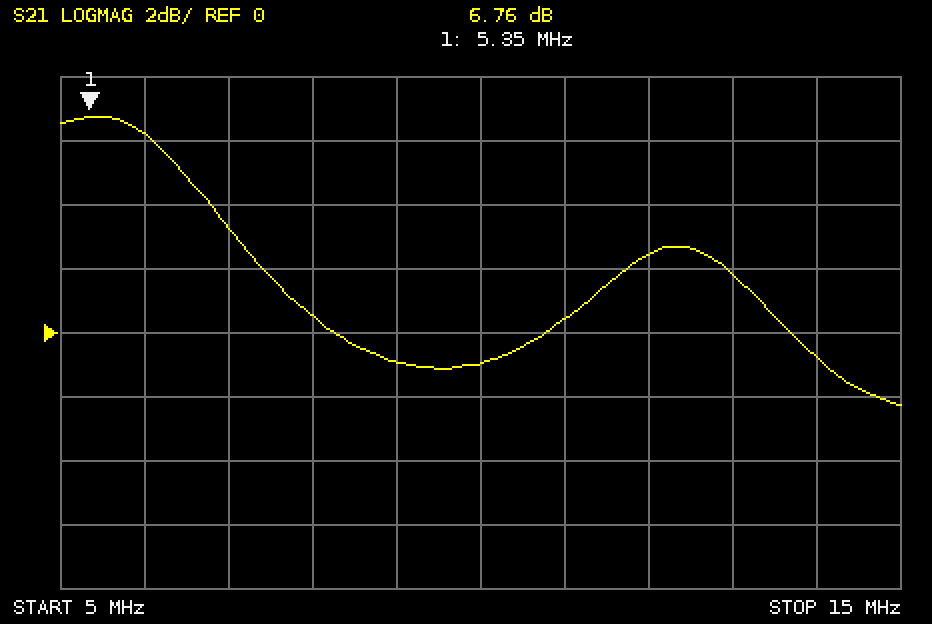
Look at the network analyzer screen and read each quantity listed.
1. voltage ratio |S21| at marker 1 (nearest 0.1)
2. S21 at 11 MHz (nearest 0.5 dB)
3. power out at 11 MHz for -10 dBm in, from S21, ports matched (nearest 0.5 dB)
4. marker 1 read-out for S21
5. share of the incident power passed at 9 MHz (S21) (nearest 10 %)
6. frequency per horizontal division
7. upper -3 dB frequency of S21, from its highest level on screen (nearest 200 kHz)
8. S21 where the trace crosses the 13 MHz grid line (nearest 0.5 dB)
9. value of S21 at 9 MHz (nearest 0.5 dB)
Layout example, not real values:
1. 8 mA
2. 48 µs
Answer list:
1. 2.2
2. 0.5 dB
3. -9.5 dBm
4. 6.76 dB
5. 80 %
6. 1 MHz
7. 6.8 MHz
8. 2.0 dB
9. -1.0 dB
